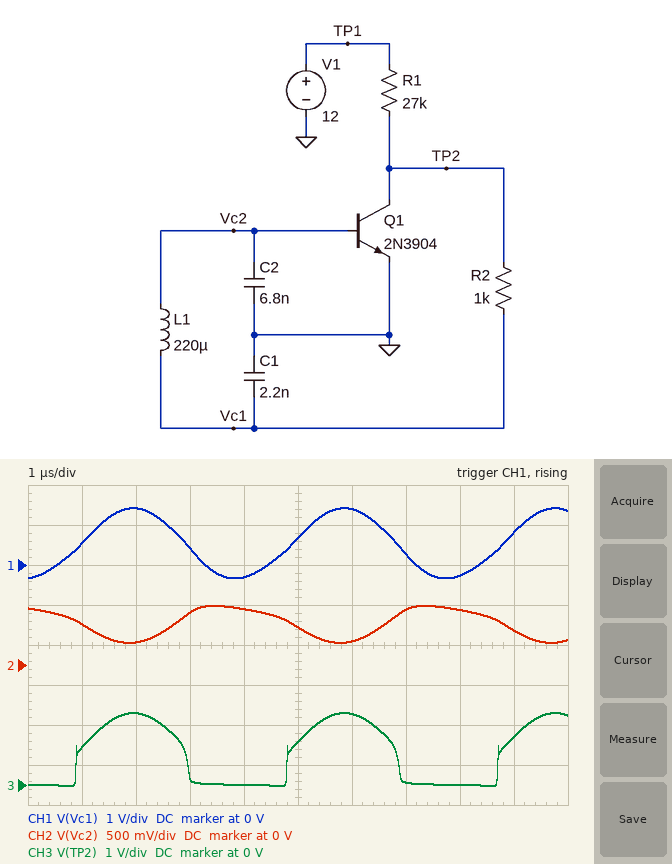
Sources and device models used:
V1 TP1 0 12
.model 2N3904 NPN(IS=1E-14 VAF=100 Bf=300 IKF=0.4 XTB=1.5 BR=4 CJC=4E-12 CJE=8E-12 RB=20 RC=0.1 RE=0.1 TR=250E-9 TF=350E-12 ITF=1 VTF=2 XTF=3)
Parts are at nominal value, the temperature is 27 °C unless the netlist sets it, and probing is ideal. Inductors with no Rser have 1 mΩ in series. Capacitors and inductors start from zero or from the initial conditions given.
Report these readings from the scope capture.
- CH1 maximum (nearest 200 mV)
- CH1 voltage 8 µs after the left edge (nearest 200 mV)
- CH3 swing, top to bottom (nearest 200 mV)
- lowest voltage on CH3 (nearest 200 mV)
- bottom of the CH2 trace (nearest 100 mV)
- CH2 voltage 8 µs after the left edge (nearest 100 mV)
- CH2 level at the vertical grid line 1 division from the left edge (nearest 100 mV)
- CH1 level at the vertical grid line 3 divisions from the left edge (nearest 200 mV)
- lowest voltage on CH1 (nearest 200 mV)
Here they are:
1.4 V
-200 mV
1.8 V
0 V
300 mV
700 mV
500 mV
400 mV
-400 mV
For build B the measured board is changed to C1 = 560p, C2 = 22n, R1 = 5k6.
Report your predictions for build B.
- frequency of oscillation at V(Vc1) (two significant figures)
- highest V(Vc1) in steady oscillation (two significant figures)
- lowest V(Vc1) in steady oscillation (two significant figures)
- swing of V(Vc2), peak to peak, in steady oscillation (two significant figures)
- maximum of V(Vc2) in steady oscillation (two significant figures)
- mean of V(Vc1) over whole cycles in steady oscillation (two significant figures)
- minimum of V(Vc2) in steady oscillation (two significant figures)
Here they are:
430 kHz
2.2 V
-750 mV
66 mV
710 mV
680 mV
650 mV
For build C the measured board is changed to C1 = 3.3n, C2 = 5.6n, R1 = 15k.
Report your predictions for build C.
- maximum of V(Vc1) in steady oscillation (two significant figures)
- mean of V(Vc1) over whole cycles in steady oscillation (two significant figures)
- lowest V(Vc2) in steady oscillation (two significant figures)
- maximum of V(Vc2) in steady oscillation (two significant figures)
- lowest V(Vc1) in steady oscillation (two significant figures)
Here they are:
1.3 V
480 mV
83 mV
770 mV
-300 mV
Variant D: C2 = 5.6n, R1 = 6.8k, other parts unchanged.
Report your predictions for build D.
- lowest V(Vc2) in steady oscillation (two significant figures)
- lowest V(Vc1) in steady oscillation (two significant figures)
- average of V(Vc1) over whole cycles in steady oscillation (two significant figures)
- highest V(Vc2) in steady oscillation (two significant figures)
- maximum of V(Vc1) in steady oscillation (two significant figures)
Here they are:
84 mV
-960 mV
520 mV
830 mV
2.1 V
